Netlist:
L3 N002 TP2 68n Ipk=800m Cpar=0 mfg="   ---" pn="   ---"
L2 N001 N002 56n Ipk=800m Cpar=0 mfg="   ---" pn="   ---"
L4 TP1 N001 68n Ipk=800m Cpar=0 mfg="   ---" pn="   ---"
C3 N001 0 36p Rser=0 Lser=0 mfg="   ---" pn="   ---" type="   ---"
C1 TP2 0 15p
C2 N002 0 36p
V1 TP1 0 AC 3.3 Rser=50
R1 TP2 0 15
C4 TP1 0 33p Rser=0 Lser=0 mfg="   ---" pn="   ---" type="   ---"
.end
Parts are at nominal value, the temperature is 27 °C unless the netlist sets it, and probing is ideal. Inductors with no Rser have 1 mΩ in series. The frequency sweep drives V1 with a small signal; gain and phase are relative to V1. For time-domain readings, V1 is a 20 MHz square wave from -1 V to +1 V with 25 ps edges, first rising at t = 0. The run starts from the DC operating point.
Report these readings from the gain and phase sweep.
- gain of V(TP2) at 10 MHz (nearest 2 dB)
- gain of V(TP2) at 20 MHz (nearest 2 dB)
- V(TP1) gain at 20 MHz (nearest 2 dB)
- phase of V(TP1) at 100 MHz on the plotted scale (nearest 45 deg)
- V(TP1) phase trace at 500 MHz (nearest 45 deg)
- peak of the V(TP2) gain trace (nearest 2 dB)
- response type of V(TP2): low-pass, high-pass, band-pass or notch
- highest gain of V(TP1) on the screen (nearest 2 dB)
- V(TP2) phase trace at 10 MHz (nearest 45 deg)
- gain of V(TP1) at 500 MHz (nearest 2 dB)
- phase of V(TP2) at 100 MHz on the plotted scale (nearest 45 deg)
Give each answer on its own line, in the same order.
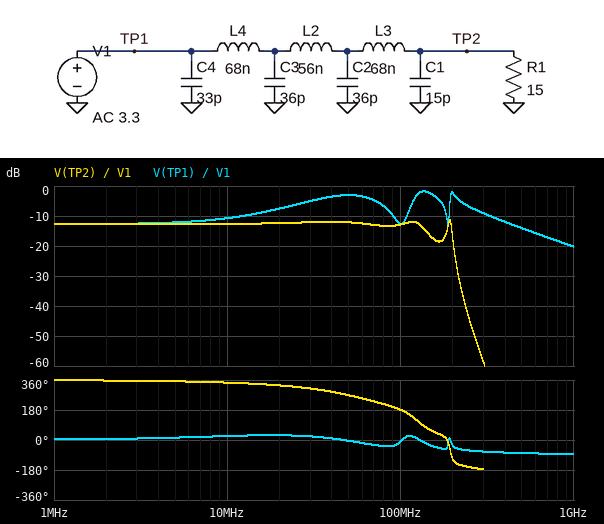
-12 dB
-12 dB
-8 dB
0 deg
-90 deg
-12 dB
low-pass
-2 dB
360 deg
-14 dB
180 deg
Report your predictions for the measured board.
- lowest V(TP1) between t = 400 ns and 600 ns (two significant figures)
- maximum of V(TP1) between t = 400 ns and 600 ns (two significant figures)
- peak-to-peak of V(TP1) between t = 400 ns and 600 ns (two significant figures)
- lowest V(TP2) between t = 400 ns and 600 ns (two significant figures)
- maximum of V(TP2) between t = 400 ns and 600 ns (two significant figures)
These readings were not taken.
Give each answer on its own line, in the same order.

-820 mV
820 mV
1.6 V
-310 mV
310 mV
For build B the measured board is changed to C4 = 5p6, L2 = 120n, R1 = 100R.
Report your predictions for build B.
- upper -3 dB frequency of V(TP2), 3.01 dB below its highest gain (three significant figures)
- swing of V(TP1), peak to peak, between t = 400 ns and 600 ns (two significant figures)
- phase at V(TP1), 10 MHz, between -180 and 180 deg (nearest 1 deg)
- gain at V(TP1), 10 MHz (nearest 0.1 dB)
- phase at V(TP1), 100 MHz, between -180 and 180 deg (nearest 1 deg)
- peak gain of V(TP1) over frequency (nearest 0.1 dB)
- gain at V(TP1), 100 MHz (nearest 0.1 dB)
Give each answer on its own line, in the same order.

136 MHz
1.7 V
-8 deg
-3.8 dB
-12 deg
0 dB
-3.6 dB
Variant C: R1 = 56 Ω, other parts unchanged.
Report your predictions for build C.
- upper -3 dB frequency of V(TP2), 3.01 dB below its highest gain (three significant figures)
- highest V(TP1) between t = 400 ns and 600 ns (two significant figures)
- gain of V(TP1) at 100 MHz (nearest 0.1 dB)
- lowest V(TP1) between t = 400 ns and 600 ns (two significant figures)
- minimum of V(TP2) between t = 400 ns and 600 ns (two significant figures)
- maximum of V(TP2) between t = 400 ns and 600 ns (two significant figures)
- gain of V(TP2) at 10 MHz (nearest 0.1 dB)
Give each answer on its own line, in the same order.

200 MHz
550 mV
-5.7 dB
-550 mV
-680 mV
680 mV
-5.6 dB
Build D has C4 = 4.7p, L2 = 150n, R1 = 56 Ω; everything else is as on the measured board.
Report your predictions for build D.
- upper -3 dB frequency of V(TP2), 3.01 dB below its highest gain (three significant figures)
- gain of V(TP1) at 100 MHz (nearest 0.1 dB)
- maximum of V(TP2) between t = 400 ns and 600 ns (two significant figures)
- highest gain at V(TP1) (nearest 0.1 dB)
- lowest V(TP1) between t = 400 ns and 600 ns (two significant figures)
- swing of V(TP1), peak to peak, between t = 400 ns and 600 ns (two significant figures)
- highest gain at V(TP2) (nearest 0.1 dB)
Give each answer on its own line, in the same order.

129 MHz
-6.0 dB
660 mV
0 dB
-1.0 V
2.1 V
-5.5 dB
